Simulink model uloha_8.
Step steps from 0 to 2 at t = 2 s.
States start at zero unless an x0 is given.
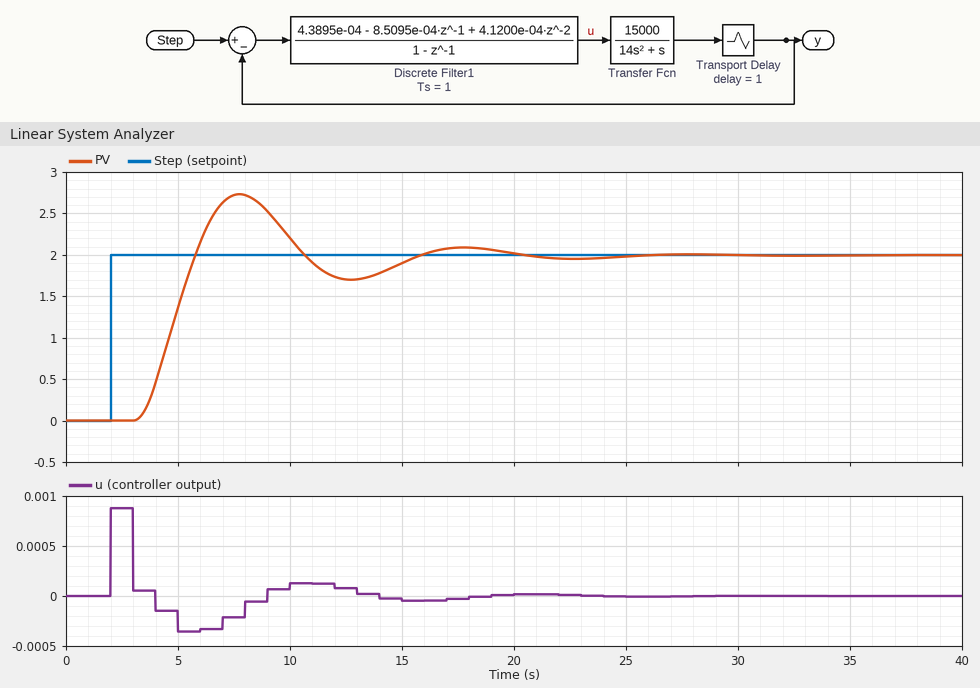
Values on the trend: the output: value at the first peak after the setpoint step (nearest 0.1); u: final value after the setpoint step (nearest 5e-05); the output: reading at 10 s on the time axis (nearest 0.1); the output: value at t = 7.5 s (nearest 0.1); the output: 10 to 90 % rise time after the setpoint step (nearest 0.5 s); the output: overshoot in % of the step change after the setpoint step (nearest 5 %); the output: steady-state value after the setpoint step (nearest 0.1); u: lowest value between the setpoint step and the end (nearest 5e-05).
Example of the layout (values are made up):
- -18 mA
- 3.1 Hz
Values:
- 2.7
- 0.00000
- 2.2
- 2.7
- 2.0 s
- 35 %
- 2.0
- -0.00035
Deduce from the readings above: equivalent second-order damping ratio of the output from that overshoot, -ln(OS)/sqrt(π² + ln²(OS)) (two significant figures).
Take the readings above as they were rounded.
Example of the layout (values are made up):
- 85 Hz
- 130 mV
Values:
- 0.32
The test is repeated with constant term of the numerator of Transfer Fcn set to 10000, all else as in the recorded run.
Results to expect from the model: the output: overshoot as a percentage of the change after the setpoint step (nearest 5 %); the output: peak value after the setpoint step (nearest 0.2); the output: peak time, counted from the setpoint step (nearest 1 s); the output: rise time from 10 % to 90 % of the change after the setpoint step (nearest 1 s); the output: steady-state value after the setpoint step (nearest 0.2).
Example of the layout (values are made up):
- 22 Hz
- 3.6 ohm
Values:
- 10 %
- 2.2
- 7 s
- 3 s
- 2.0
